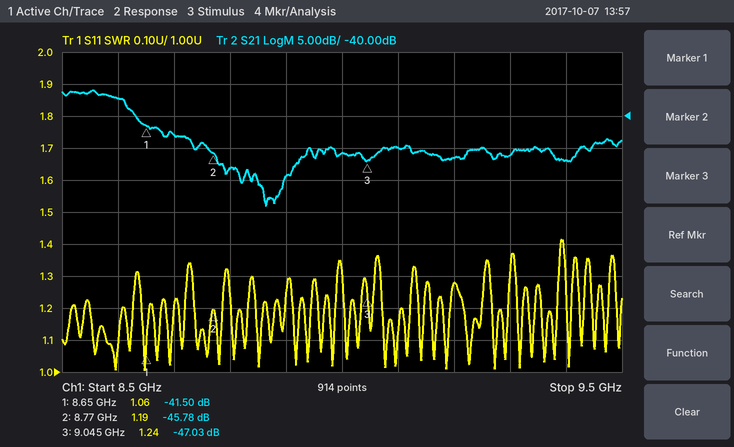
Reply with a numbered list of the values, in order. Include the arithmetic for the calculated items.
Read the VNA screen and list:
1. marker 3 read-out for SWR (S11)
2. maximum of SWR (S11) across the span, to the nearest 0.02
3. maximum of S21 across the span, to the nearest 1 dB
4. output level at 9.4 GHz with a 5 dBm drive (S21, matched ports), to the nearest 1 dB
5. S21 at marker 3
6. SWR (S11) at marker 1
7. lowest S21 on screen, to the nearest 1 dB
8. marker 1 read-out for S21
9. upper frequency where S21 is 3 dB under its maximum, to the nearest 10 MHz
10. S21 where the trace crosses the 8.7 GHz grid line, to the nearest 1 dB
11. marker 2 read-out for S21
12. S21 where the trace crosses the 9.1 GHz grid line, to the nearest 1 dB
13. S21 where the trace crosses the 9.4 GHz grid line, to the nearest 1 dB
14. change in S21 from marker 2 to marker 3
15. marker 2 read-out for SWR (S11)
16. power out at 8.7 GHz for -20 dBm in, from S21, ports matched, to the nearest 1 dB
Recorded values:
1. 1.24
2. 1.42
3. -36 dB
4. 5 dBm + (-47 dB) = -42 dBm
5. -47.03 dB
6. 1.06
7. -54 dB
8. -41.50 dB
9. 8.62 GHz
10. -43 dB
11. -45.78 dB
12. -45 dB
13. -47 dB
14. -47.03 − (-45.78) = -1.25 dB
15. 1.19
16. -20 dBm + (-43 dB) = -63 dBm
